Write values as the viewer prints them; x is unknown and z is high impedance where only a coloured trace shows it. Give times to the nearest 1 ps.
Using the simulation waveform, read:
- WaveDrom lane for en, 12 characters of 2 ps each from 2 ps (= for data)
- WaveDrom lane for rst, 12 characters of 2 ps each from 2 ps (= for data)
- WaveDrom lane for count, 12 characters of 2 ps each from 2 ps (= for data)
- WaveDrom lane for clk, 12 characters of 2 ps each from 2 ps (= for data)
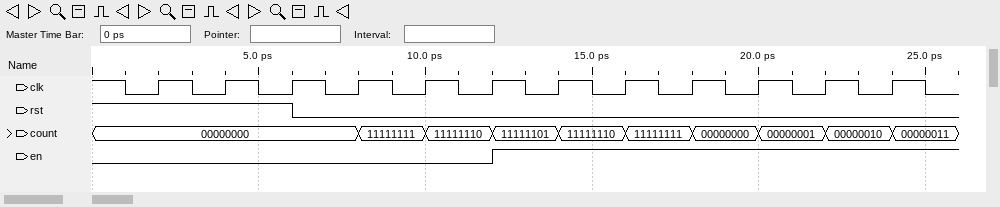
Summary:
{name: 'en', wave: '0....1......'}
{name: 'rst', wave: '1.0.........'}
{name: 'count', wave: '=..=========', data: '00000000 11111111 11111110 11111101 11111110 11111111 00000000 00000001 00000010 00000011'}
{name: 'clk', wave: 'p...........'}
